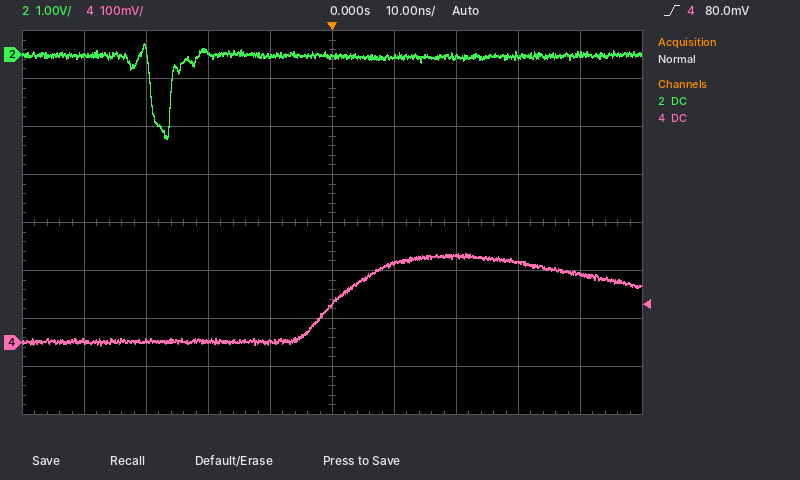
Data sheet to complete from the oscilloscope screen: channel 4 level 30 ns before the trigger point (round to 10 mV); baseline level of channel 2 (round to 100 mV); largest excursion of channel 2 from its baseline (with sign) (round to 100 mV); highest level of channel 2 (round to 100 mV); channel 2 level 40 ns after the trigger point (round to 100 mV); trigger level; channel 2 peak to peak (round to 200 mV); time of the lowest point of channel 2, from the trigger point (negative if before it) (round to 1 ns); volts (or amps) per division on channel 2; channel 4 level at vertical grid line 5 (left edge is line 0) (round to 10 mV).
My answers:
0 mV
0.0 V
-1.7 V
200 mV
0.0 V
80.0 mV
2.0 V
-27 ns
1 V
80 mV
